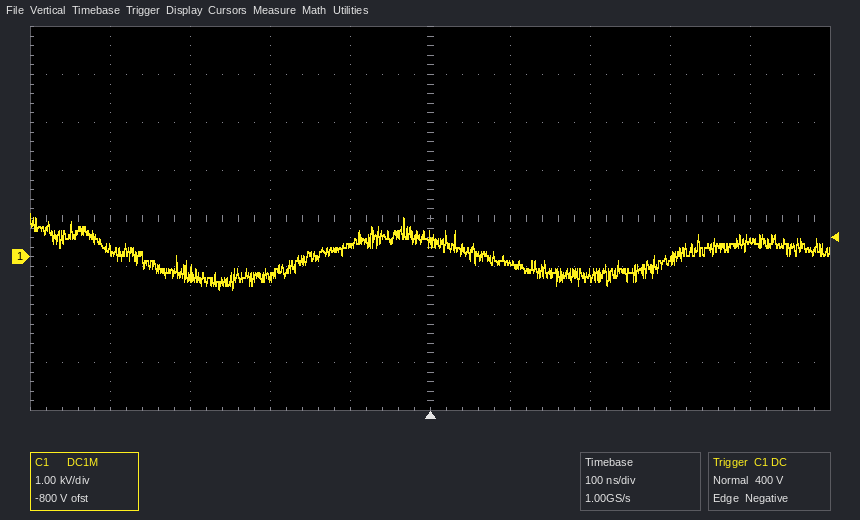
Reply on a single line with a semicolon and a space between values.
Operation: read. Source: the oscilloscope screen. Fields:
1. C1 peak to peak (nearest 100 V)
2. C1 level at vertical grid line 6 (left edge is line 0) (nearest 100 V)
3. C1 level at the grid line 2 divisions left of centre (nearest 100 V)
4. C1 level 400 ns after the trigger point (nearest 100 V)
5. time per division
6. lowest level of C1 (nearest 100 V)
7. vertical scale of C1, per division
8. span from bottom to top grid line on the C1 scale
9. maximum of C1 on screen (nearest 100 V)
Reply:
1.6 kV; -100 V; -400 V; 400 V; 100 ns; -700 V; 1 kV; 8 kV; 900 V
